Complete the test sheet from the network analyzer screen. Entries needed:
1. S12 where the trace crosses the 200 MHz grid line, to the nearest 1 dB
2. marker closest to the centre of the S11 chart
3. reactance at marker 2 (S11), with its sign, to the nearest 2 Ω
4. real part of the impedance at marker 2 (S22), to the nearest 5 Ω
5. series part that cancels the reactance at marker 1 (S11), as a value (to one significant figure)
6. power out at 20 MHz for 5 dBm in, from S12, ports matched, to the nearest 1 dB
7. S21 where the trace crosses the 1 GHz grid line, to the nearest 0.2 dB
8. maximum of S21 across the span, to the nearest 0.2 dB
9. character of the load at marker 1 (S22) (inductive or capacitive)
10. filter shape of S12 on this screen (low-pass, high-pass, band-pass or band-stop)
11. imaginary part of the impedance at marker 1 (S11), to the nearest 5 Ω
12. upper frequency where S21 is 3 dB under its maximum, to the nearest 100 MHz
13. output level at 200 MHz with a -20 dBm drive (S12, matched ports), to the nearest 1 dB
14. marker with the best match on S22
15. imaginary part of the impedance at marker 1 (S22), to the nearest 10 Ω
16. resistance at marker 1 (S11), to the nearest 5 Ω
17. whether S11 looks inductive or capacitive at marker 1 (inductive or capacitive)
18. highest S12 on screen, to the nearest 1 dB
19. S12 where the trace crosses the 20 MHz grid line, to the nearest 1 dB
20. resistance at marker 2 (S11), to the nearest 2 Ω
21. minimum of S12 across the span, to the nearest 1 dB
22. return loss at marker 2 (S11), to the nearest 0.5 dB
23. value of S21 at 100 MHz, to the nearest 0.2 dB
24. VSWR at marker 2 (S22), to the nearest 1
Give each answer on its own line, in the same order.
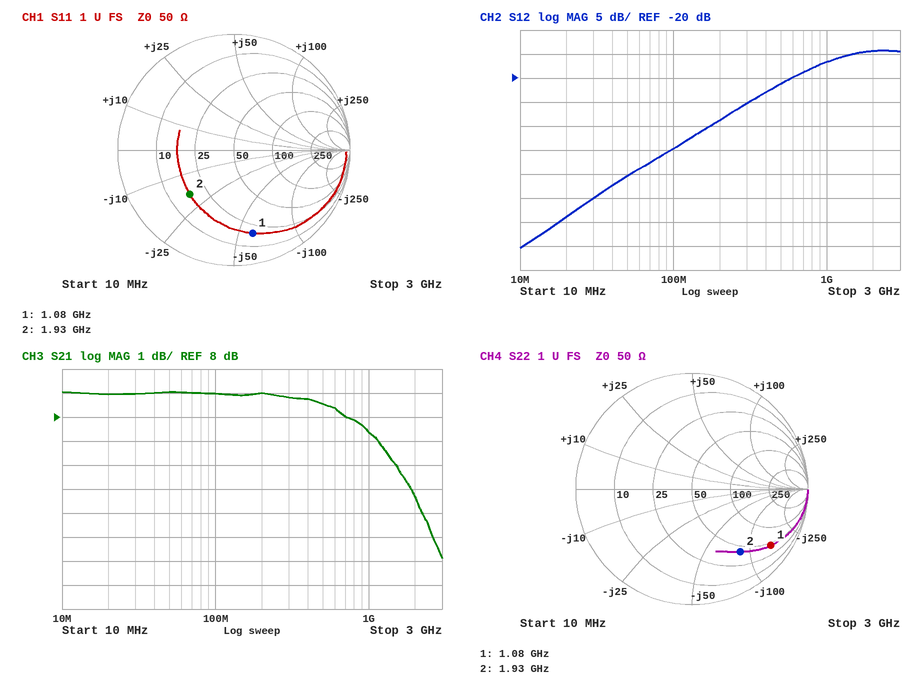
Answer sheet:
-29 dB
marker 2
-18 Ω
40 Ω
9 nH
-44 dBm
7.4 dB
9.0 dB
capacitive
high-pass
-60 Ω
1.5 GHz
-49 dBm
marker 2
-140 Ω
20 Ω
capacitive
-14 dB
-49 dB
18 Ω
-55 dB
5.5 dB
9.0 dB
5
